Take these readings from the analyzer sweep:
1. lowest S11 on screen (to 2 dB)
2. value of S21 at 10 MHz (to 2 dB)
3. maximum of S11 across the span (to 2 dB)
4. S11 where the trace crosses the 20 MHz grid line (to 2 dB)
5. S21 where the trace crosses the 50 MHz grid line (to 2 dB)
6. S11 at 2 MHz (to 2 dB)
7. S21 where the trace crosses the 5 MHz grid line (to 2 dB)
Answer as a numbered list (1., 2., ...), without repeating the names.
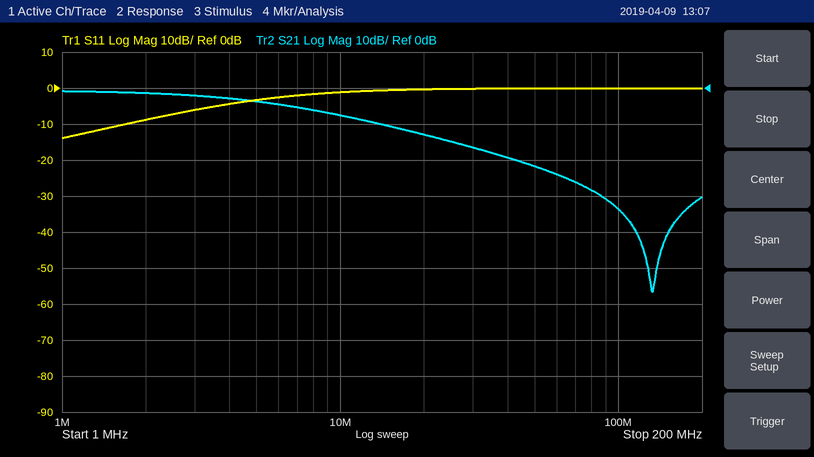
1. -14 dB
2. -8 dB
3. 0 dB
4. 0 dB
5. -22 dB
6. -8 dB
7. -4 dB
